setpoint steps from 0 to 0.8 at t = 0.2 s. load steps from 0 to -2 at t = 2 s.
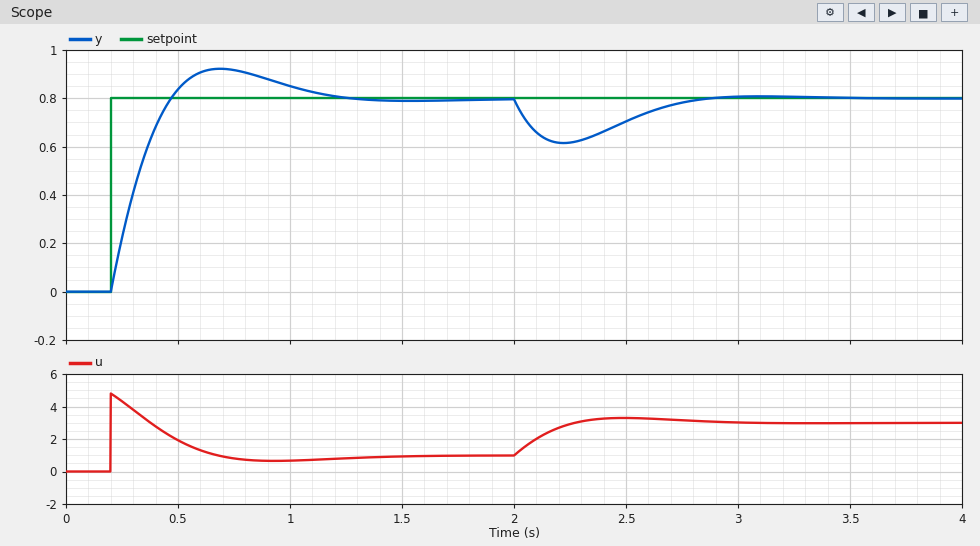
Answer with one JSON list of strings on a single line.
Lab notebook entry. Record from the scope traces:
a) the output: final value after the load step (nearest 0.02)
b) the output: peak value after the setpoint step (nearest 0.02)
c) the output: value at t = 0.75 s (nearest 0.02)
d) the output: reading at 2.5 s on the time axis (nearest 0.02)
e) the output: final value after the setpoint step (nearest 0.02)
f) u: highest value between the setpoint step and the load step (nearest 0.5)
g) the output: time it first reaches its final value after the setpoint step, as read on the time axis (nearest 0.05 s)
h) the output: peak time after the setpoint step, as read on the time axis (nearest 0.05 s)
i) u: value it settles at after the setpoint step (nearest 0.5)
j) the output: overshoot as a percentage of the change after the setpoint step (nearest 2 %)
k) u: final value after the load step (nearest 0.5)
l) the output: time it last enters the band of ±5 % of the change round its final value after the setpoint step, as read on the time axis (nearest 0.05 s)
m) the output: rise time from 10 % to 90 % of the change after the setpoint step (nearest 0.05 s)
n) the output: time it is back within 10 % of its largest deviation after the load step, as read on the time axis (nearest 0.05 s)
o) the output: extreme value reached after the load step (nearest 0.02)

["0.80", "0.92", "0.92", "0.70", "0.80", "5.0", "0.45 s", "0.70 s", "1.0", "16 %", "3.0", "1.05 s", "0.20 s", "2.75 s", "0.62"]
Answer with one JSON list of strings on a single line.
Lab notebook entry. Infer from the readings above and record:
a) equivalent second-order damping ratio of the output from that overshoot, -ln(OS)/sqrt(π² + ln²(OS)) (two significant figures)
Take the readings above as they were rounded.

["0.50"]
